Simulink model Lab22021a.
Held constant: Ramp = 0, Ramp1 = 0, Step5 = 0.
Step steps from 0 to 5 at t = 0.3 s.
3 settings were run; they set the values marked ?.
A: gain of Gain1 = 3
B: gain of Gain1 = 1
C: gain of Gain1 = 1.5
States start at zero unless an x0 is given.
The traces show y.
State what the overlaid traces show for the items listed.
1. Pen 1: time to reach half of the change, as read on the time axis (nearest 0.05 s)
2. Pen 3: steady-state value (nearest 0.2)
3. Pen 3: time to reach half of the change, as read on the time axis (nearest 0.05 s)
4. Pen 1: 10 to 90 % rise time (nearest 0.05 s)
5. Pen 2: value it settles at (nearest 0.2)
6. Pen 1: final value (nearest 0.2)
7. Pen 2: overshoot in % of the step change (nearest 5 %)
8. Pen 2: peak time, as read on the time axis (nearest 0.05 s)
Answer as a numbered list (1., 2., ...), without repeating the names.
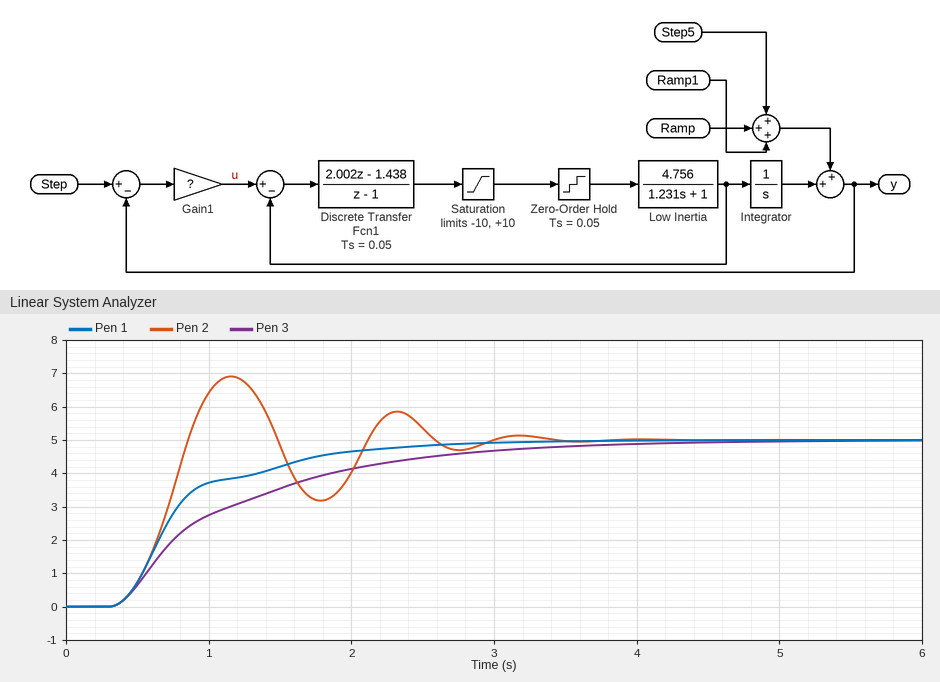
1. 0.70 s
2. 5.0
3. 0.90 s
4. 1.30 s
5. 5.0
6. 5.0
7. 40 %
8. 1.15 s
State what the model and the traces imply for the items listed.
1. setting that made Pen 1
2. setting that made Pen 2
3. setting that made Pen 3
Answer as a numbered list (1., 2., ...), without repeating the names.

1. C
2. A
3. B
